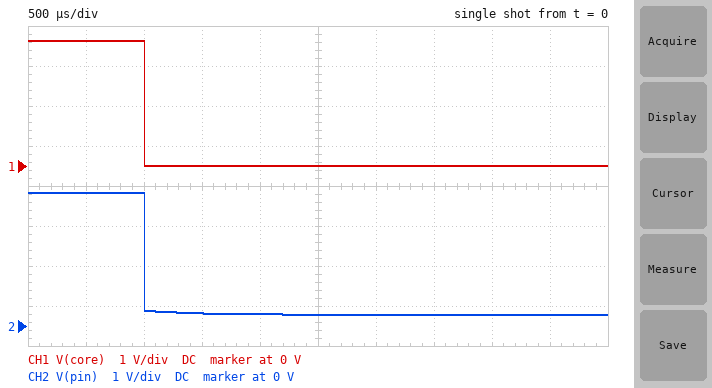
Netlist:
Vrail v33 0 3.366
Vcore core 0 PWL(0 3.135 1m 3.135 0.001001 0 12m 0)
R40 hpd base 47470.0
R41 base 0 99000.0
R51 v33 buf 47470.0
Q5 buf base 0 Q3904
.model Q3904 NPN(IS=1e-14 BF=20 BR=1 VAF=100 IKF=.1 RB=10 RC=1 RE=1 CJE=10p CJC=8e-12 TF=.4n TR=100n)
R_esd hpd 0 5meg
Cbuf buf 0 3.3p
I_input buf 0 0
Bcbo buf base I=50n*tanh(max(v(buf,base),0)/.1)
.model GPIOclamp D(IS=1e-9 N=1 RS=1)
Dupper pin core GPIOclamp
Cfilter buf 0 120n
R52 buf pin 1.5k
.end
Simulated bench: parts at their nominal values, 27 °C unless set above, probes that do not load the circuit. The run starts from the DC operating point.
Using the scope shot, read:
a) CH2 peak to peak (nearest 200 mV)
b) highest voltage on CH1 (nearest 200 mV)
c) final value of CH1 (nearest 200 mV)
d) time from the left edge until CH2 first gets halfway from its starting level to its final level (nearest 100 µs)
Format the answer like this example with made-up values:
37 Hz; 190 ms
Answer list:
3.0 V; 3.2 V; 0 V; 1.0 ms
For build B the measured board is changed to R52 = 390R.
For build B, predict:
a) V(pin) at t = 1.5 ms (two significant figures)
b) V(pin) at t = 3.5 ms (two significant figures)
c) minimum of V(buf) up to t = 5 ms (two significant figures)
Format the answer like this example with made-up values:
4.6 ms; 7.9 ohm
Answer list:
290 mV; 290 mV; 310 mV
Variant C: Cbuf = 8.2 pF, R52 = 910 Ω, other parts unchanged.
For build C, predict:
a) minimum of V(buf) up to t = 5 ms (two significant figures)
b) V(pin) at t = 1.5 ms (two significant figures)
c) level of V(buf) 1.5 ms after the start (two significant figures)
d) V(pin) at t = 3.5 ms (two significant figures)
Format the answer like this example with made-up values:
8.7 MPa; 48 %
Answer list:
340 mV; 300 mV; 400 mV; 290 mV
